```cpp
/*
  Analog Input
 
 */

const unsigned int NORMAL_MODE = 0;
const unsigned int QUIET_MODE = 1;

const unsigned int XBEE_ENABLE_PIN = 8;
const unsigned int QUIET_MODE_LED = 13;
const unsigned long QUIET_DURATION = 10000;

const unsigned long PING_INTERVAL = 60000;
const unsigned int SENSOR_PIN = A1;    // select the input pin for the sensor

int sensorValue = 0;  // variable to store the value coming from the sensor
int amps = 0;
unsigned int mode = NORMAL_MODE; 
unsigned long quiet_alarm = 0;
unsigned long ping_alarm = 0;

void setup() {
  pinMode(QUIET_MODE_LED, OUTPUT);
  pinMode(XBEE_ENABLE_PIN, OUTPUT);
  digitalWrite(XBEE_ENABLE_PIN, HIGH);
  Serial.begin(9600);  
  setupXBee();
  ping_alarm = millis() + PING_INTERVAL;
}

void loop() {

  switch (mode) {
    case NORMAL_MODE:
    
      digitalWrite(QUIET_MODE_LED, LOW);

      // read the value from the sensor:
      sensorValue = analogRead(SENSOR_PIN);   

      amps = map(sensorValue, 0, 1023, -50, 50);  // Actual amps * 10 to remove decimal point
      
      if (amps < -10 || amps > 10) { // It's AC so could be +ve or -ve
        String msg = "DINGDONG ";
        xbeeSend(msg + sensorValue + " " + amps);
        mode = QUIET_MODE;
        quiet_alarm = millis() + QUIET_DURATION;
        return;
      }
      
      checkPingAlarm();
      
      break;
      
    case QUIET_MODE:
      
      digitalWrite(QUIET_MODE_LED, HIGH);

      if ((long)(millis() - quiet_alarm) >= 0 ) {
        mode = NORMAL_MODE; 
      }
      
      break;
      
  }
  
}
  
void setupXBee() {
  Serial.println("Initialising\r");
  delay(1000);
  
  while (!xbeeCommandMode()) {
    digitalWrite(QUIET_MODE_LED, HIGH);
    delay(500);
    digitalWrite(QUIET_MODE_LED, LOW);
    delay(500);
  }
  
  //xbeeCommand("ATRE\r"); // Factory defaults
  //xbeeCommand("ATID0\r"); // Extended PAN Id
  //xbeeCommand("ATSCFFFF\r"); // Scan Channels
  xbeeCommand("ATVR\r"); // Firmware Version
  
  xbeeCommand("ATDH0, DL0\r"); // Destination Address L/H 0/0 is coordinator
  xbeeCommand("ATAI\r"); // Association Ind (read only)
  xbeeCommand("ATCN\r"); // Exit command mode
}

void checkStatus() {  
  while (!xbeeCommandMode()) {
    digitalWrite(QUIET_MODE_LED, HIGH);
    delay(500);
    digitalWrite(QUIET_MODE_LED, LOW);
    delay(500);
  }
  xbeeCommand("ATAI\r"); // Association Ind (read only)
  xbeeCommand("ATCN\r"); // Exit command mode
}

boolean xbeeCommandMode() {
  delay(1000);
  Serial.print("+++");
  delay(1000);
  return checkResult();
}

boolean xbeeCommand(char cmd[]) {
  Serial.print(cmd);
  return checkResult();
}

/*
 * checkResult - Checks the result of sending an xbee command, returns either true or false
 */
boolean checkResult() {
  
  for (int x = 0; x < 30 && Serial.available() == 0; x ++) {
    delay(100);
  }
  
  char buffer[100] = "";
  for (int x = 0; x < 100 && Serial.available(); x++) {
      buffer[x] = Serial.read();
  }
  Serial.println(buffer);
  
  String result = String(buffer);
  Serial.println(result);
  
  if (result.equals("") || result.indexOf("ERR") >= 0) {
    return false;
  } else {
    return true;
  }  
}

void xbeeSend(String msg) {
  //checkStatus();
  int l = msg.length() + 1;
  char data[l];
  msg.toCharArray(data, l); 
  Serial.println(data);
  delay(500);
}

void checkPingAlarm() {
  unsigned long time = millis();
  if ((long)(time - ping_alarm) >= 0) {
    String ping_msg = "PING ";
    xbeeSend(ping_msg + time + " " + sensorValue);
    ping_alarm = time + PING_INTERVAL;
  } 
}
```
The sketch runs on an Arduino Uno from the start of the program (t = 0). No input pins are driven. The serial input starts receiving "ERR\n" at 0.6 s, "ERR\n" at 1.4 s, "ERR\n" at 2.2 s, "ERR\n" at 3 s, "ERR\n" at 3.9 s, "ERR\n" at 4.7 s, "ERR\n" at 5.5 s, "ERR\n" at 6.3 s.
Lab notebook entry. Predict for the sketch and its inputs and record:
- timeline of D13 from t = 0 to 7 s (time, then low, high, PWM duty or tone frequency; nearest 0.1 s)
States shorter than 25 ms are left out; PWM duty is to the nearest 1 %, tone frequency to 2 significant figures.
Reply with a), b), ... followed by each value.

a) 0 s low; 3 s high; 3.5 s low; 6 s high; 6.5 s low
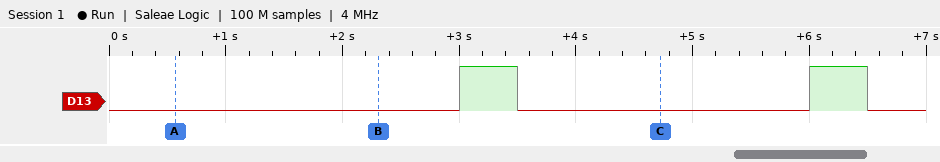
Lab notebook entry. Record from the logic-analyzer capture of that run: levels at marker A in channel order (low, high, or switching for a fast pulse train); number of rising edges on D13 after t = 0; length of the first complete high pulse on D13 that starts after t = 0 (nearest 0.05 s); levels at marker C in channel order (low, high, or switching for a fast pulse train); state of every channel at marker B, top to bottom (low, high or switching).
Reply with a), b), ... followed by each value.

a) D13 low
b) 2
c) 0.50 s
d) D13 low
e) D13 low
